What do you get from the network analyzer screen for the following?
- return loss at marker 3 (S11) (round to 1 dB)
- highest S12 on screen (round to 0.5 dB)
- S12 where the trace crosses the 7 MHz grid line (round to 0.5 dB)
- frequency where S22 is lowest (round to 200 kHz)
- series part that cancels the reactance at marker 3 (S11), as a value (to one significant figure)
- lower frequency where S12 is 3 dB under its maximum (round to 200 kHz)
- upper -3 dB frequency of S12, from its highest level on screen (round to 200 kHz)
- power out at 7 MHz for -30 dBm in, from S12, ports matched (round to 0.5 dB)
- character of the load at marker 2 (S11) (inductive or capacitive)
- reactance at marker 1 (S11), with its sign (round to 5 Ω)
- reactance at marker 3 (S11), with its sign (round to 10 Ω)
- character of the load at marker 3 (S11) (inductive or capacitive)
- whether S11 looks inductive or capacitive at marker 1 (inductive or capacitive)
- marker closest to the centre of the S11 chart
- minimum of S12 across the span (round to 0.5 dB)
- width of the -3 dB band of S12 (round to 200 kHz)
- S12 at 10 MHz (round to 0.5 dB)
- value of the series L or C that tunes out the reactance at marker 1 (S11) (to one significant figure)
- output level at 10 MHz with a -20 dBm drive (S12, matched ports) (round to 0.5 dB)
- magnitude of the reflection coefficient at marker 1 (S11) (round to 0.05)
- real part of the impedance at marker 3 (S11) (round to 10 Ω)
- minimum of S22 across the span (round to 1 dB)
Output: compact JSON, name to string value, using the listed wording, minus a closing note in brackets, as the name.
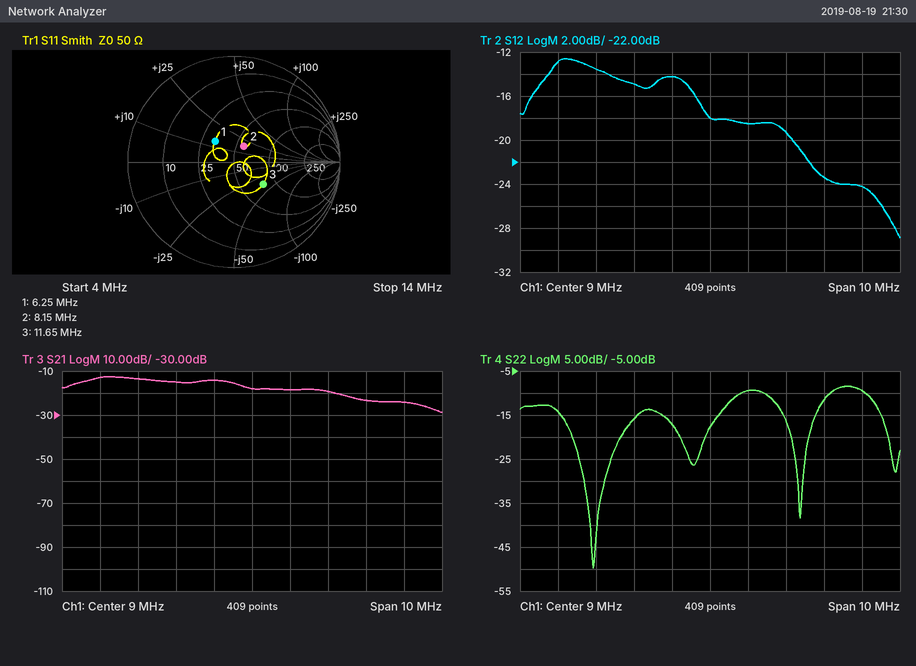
{"return loss at marker 3 (S11)": "9 dB", "highest S12 on screen": "-12.5 dB", "S12 where the trace crosses the 7 MHz grid line": "-15.0 dB", "frequency where S22 is lowest": "6.0 MHz", "series part that cancels the reactance at marker 3 (S11), as a value": "500 nH", "lower frequency where S12 is 3 dB under its maximum": "4.4 MHz", "upper -3 dB frequency of S12, from its highest level on screen": "8.6 MHz", "power out at 7 MHz for -30 dBm in, from S12, ports matched": "-45.0 dBm", "character of the load at marker 2 (S11)": "inductive", "reactance at marker 1 (S11), with its sign": "+15 Ω", "reactance at marker 3 (S11), with its sign": "-40 Ω", "character of the load at marker 3 (S11)": "capacitive", "whether S11 looks inductive or capacitive at marker 1": "inductive", "marker closest to the centre of the S11 chart": "marker 2", "minimum of S12 across the span": "-29.0 dB", "width of the -3 dB band of S12": "4.2 MHz", "S12 at 10 MHz": "-18.5 dB", "value of the series L or C that tunes out the reactance at marker 1 (S11)": "2 nF", "output level at 10 MHz with a -20 dBm drive (S12, matched ports)": "-38.5 dBm", "magnitude of the reflection coefficient at marker 1 (S11)": "0.25", "real part of the impedance at marker 3 (S11)": "80 Ω", "minimum of S22 across the span": "-50 dB"}
